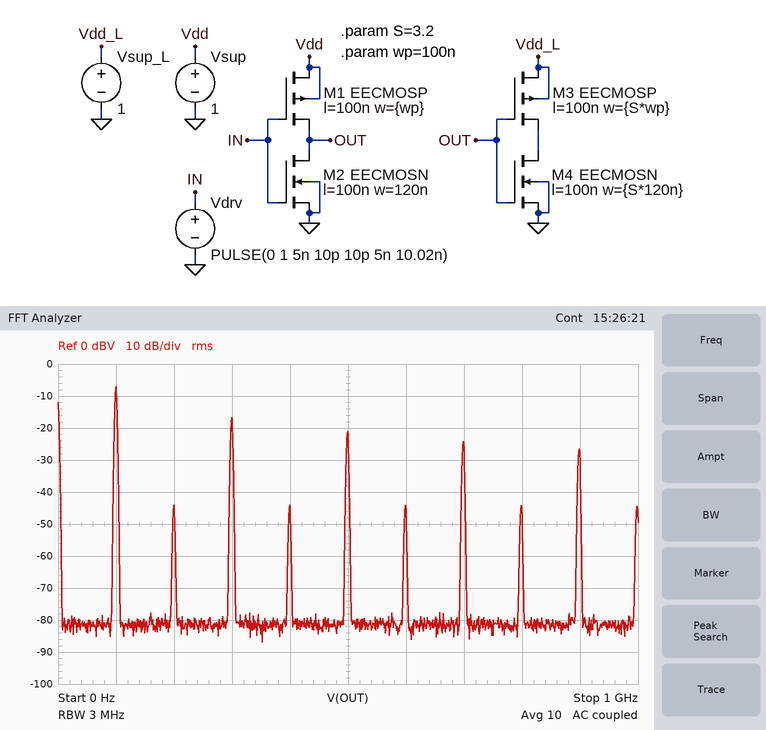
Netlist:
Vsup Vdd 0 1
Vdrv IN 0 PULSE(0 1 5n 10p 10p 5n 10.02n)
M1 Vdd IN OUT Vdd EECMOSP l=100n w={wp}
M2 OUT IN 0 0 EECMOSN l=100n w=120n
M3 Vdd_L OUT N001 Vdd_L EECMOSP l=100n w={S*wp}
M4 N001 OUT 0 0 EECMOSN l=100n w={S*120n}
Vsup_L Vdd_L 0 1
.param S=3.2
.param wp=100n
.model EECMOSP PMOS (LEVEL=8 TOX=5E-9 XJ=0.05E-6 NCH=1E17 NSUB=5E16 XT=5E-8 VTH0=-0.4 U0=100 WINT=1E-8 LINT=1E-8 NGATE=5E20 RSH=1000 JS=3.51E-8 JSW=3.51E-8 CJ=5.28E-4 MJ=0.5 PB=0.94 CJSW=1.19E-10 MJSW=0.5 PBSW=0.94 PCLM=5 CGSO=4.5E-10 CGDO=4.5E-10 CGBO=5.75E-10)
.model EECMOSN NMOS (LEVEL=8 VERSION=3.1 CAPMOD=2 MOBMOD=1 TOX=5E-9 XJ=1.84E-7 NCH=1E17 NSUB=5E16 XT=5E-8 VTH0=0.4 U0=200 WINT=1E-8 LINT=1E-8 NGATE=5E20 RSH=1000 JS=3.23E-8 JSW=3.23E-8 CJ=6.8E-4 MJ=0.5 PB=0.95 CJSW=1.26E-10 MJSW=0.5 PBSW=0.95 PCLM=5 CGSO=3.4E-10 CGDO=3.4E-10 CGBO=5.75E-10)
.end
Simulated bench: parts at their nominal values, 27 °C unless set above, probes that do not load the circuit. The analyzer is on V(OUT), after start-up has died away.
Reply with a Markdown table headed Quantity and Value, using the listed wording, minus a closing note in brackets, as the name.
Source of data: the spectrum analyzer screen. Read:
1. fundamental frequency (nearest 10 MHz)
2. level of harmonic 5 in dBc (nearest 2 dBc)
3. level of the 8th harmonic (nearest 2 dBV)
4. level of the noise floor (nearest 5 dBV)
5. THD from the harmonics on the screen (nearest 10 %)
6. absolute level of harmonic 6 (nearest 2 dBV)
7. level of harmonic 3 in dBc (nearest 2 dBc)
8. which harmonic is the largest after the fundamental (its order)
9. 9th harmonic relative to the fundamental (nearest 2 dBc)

| Quantity | Value |
|---|---|
| fundamental frequency | 100 MHz |
| level of harmonic 5 in dBc | -14 dBc |
| level of the 8th harmonic | -44 dBV |
| level of the noise floor | -80 dBV |
| THD from the harmonics on the screen | 40 % |
| absolute level of harmonic 6 | -44 dBV |
| level of harmonic 3 in dBc | -10 dBc |
| which harmonic is the largest after the fundamental | 3 |
| 9th harmonic relative to the fundamental | -20 dBc |
